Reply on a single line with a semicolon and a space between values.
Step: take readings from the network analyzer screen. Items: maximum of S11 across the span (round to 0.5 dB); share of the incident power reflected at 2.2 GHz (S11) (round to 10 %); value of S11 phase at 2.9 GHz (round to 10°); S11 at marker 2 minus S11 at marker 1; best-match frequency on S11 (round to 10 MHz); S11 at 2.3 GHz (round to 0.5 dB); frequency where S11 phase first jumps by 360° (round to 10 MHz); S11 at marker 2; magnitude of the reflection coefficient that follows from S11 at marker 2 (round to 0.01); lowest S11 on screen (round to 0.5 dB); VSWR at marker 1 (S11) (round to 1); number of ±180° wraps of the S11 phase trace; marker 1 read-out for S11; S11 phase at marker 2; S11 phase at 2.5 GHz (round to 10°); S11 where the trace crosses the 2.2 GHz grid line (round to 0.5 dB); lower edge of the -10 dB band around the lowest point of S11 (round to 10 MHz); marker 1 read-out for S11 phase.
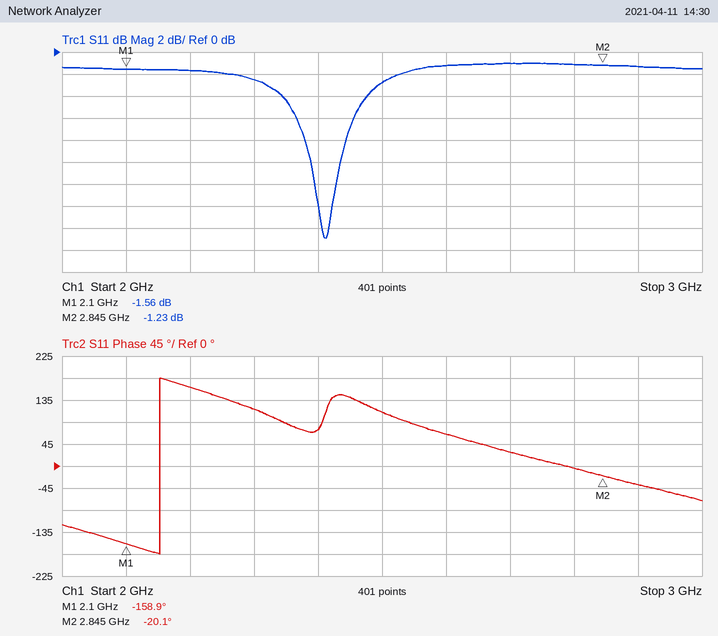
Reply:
-1.0 dB; 70 %; -40°; 0.33 dB; 2.41 GHz; -2.5 dB; 2.15 GHz; -1.23 dB; 0.87; -17.0 dB; 11; 1; -1.56 dB; -20.1°; 110°; -1.5 dB; 2.39 GHz; -158.9°
